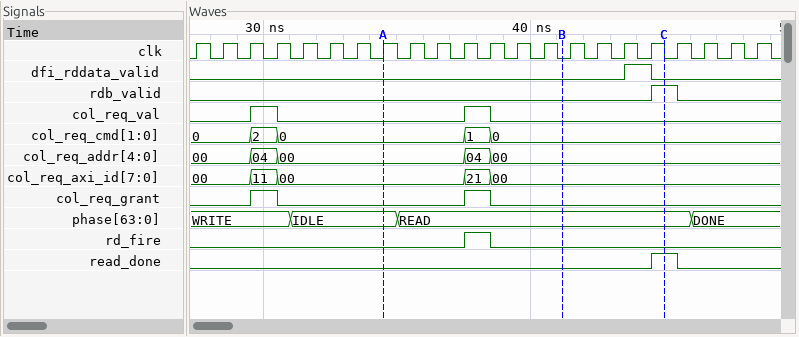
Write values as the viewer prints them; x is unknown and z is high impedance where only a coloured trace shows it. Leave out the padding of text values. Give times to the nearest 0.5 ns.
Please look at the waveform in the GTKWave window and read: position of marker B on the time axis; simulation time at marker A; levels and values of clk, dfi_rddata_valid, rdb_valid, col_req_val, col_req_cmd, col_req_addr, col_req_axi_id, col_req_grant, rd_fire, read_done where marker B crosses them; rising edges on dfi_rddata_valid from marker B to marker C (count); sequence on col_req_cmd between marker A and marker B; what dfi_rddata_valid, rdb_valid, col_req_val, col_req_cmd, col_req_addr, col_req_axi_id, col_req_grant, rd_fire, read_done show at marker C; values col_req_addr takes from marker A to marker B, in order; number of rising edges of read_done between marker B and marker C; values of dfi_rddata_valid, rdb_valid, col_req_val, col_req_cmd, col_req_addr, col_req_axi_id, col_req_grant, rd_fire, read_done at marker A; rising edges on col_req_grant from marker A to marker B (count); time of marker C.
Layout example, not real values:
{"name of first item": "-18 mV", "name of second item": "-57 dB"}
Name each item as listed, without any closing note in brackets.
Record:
{"position of marker B on the time axis": "41 ns", "simulation time at marker A": "34.5 ns", "levels and values of clk, dfi_rddata_valid, rdb_valid, col_req_val, col_req_cmd, col_req_addr, col_req_axi_id, col_req_grant, rd_fire, read_done where marker B crosses them": "clk=0, dfi_rddata_valid=0, rdb_valid=0, col_req_val=0, col_req_cmd=0, col_req_addr=00, col_req_axi_id=00, col_req_grant=0, rd_fire=0, read_done=0", "rising edges on dfi_rddata_valid from marker B to marker C": "1", "sequence on col_req_cmd between marker A and marker B": "0, 1, 0", "what dfi_rddata_valid, rdb_valid, col_req_val, col_req_cmd, col_req_addr, col_req_axi_id, col_req_grant, rd_fire, read_done show at marker C": "dfi_rddata_valid=0, rdb_valid=1, col_req_val=0, col_req_cmd=0, col_req_addr=00, col_req_axi_id=00, col_req_grant=0, rd_fire=0, read_done=1", "values col_req_addr takes from marker A to marker B, in order": "00, 04, 00", "number of rising edges of read_done between marker B and marker C": "1", "values of dfi_rddata_valid, rdb_valid, col_req_val, col_req_cmd, col_req_addr, col_req_axi_id, col_req_grant, rd_fire, read_done at marker A": "dfi_rddata_valid=0, rdb_valid=0, col_req_val=0, col_req_cmd=0, col_req_addr=00, col_req_axi_id=00, col_req_grant=0, rd_fire=0, read_done=0", "rising edges on col_req_grant from marker A to marker B": "1", "time of marker C": "45 ns"}
